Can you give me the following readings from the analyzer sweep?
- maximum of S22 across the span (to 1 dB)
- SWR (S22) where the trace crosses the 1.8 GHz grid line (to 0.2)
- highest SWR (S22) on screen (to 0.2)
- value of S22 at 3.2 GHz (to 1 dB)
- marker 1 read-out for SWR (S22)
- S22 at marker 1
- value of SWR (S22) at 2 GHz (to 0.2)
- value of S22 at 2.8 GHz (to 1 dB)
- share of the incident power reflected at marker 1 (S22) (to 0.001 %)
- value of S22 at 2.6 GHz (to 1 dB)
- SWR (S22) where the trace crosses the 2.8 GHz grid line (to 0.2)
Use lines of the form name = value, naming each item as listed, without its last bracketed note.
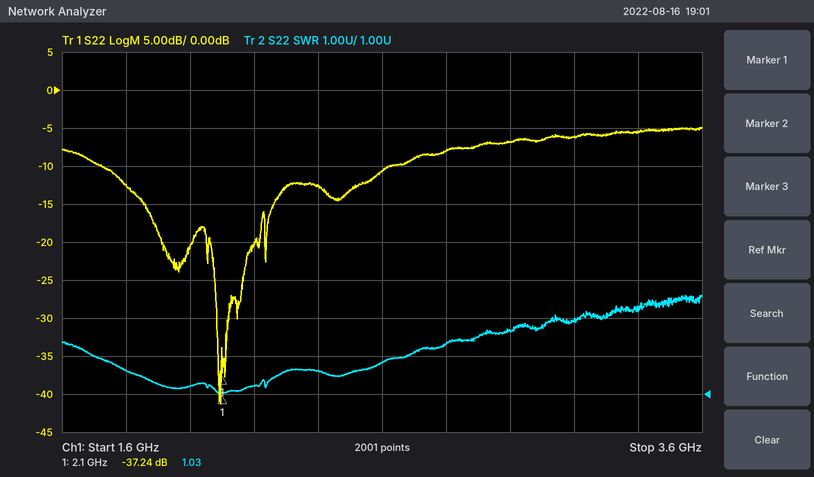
maximum of S22 across the span = -5 dB
SWR (S22) where the trace crosses the 1.8 GHz grid line = 1.6
highest SWR (S22) on screen = 3.6
value of S22 at 3.2 GHz = -6 dB
marker 1 read-out for SWR = 1.03
S22 at marker 1 = -37.24 dB
value of SWR (S22) at 2 GHz = 1.2
value of S22 at 2.8 GHz = -8 dB
share of the incident power reflected at marker 1 (S22) = 0.019 %
value of S22 at 2.6 GHz = -11 dB
SWR (S22) where the trace crosses the 2.8 GHz grid line = 2.4
